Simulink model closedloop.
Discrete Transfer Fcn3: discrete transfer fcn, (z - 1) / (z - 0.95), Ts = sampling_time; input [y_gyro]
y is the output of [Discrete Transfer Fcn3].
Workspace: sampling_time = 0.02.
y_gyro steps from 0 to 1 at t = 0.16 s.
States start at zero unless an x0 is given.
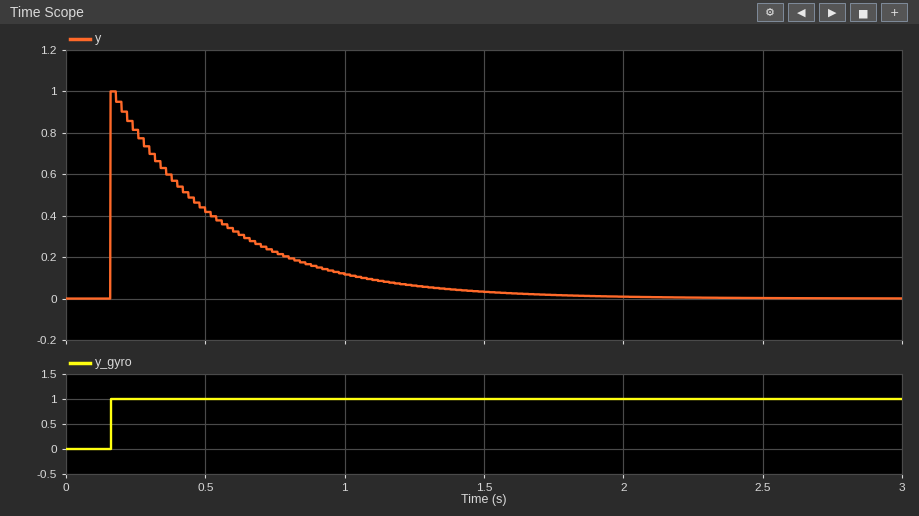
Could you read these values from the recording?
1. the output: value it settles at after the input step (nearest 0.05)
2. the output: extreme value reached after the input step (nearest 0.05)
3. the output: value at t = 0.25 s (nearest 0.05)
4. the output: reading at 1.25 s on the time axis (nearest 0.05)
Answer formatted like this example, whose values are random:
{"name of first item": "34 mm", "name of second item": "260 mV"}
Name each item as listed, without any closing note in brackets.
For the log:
{"the output: value it settles at after the input step": "0.00", "the output: extreme value reached after the input step": "1.00", "the output: value at t = 0.25 s": "0.80", "the output: reading at 1.25 s on the time axis": "0.05"}
